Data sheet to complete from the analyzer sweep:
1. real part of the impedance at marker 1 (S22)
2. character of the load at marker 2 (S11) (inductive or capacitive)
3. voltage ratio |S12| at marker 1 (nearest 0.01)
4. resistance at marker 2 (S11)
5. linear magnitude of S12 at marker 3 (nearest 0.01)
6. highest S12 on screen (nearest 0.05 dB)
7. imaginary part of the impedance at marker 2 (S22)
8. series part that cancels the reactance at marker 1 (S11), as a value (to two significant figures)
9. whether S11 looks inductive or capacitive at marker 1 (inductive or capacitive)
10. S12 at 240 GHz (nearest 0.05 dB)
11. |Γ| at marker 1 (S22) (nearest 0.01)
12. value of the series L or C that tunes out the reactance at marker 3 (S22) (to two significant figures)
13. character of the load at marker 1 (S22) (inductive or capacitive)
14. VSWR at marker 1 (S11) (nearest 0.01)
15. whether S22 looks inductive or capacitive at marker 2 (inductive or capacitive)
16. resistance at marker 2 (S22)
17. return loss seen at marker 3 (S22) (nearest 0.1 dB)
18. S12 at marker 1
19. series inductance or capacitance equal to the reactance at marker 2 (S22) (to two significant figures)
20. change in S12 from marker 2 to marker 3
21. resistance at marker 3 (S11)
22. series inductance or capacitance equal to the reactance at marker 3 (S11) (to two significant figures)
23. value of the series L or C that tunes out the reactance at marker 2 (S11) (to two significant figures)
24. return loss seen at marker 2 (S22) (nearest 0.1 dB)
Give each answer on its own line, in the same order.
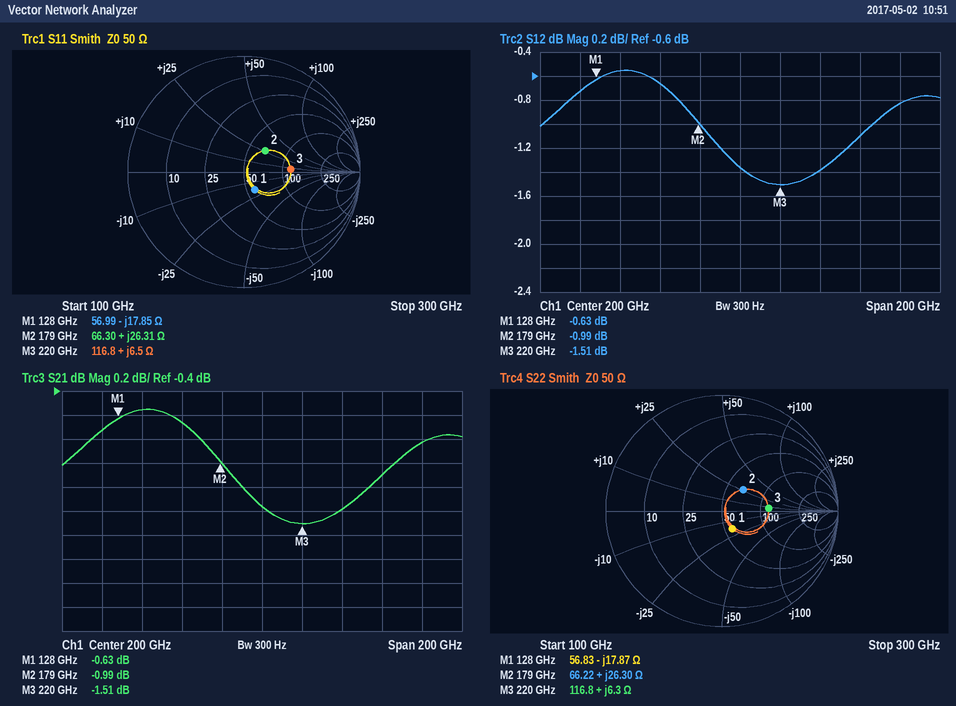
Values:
56.83 Ω
inductive
0.93
66.30 Ω
0.84
-0.55 dB
+26.30 Ω
22 pH
capacitive
-1.40 dB
0.18
110 fF
capacitive
1.43
inductive
66.22 Ω
7.9 dB
-0.63 dB
23 pH
-0.52 dB
116.8 Ω
4.7 pH
34 fF
11.7 dB
